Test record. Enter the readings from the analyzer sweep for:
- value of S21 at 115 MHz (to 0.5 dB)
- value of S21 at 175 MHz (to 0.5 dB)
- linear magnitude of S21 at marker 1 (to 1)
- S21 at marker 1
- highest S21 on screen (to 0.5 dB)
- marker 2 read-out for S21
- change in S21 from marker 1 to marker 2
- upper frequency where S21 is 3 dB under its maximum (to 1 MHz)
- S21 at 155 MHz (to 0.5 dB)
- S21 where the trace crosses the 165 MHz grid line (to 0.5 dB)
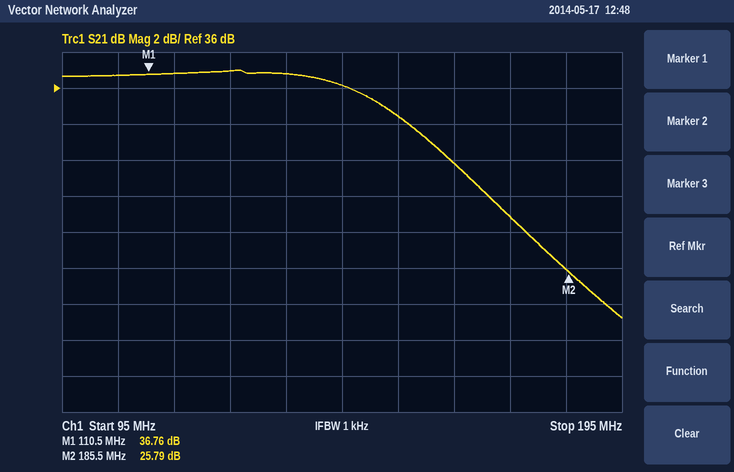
37.0 dB
29.0 dB
69
36.76 dB
37.0 dB
25.79 dB
-10.97 dB
157 MHz
34.5 dB
32.0 dB
